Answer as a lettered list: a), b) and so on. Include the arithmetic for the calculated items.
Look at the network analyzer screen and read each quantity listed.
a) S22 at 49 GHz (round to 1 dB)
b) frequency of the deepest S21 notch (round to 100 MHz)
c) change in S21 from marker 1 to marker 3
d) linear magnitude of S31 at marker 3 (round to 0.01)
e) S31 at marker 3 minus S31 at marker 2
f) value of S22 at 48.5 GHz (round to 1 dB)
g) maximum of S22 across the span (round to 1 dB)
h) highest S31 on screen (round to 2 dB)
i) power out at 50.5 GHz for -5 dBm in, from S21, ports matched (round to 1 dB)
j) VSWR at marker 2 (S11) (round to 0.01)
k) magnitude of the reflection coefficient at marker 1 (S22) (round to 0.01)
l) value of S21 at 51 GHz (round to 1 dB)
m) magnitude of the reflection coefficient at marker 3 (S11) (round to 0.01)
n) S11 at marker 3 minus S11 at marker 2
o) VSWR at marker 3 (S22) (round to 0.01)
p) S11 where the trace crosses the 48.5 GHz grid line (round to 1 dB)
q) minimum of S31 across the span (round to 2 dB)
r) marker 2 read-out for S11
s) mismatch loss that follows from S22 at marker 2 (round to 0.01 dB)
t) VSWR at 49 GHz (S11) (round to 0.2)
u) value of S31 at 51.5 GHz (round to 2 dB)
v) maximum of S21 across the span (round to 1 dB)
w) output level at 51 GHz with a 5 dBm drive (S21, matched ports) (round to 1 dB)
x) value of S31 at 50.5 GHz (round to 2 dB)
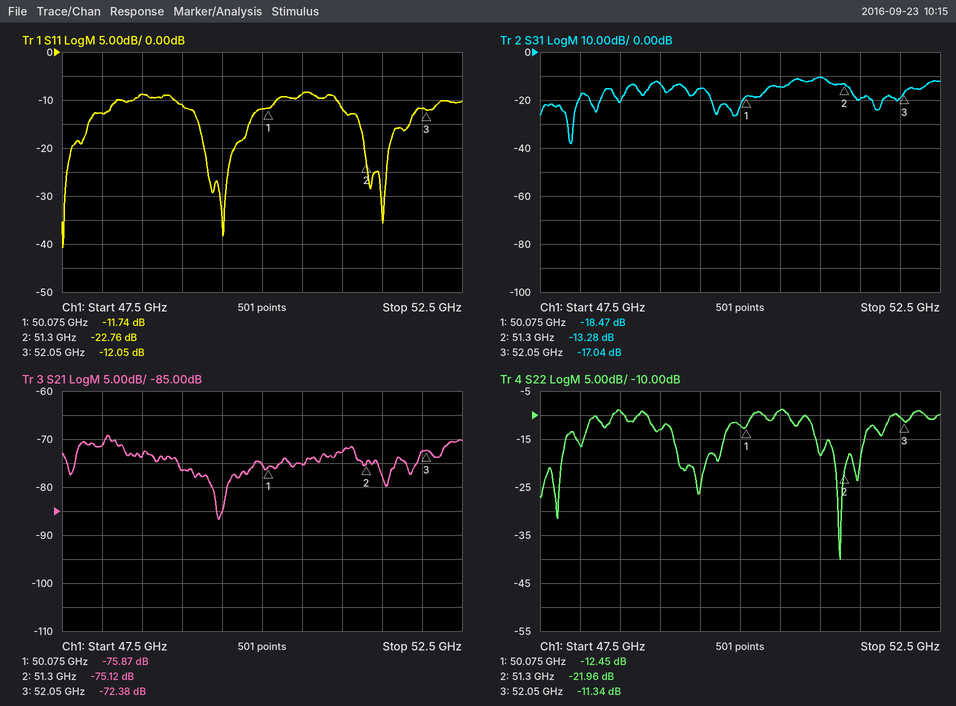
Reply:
a) -13 dB
b) 49.5 GHz
c) -72.38 − (-75.87) = 3.49 dB
d) 10^(-17.04/20) ≈ 0.14
e) -17.04 − (-13.28) = -3.76 dB
f) -9 dB
g) -9 dB
h) -10 dB
i) -5 dBm + (-75 dB) = -80 dBm
j) (1 + 0.0728)/(1 − 0.0728) ≈ 1.16
k) 10^(-12.45/20) ≈ 0.24
l) -73 dB
m) 10^(-12.05/20) ≈ 0.25
n) -12.05 − (-22.76) = 10.71 dB
o) (1 + 0.2710)/(1 − 0.2710) ≈ 1.74
p) -9 dB
q) -38 dB
r) -22.76 dB
s) −10 log10(1 − 10^(-21.96/10)) ≈ 0.03 dB
t) |Γ| = 10^(-11/20) = 0.2818; VSWR = (1 + 0.2818)/(1 − 0.2818) ≈ 1.8
u) -20 dB
v) -69 dB
w) 5 dBm + (-73 dB) = -68 dBm
x) -14 dB
